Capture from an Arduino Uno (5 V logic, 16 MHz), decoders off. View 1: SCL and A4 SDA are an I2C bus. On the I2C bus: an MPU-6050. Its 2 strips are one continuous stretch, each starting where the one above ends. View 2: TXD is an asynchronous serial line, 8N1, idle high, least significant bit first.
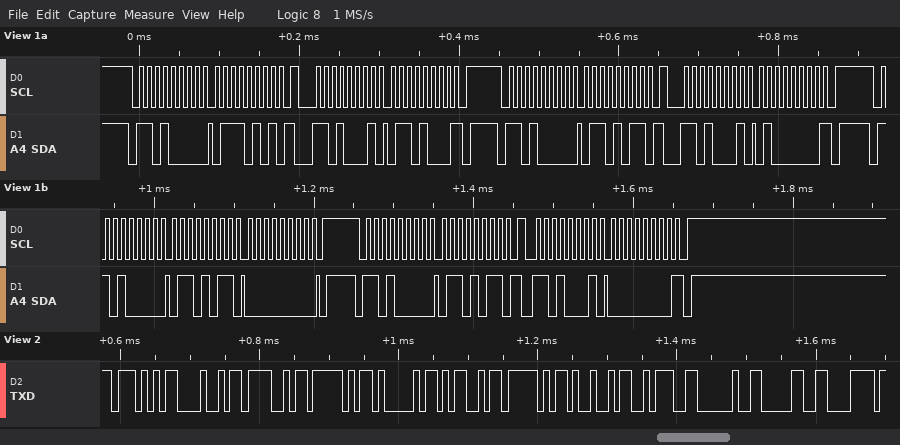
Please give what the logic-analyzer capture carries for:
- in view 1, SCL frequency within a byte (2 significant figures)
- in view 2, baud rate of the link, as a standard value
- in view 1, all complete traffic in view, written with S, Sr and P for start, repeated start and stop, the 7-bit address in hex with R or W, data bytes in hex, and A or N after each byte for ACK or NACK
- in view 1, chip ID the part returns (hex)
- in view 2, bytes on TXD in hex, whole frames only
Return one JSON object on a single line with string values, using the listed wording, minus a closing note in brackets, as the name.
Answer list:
{"in view 1, SCL frequency within a byte": "100 kHz", "in view 2, baud rate of the link, as a standard value": "115200 baud", "in view 1, all complete traffic in view, written with S, Sr and P for start, repeated start and stop, the 7-bit address in hex with R or W, data bytes in hex, and A or N after each byte for ACK or NACK": "S 68W A 75 A Sr 68R A 68 N P S 68W A 6B A Sr 68R A 40 N P S 68W A 6B A 00 A P S 68W A 6B A Sr 68R A 00 N P", "in view 1, chip ID the part returns": "0x68", "in view 2, bytes on TXD in hex, whole frames only": "57 48 4F 5F 41 4D 5F 49 3A 20 30 78"}
